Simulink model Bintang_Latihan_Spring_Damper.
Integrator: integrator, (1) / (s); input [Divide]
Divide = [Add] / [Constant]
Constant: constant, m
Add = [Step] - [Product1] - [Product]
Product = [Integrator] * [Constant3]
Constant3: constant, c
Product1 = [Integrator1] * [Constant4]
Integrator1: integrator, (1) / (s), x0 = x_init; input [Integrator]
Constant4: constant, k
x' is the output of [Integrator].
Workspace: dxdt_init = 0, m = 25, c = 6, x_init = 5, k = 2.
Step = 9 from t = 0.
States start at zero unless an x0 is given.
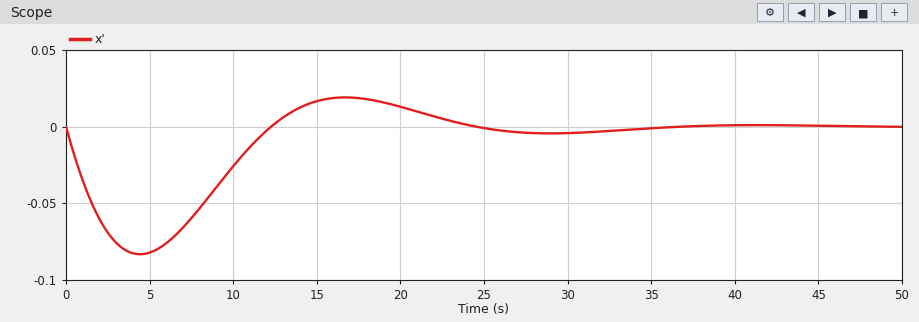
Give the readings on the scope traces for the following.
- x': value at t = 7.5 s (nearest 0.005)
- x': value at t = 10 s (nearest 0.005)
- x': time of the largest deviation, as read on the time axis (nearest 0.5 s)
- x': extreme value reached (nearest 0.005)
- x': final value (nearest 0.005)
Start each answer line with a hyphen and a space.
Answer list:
- -0.060
- -0.025
- 4.5 s
- -0.085
- 0.000
